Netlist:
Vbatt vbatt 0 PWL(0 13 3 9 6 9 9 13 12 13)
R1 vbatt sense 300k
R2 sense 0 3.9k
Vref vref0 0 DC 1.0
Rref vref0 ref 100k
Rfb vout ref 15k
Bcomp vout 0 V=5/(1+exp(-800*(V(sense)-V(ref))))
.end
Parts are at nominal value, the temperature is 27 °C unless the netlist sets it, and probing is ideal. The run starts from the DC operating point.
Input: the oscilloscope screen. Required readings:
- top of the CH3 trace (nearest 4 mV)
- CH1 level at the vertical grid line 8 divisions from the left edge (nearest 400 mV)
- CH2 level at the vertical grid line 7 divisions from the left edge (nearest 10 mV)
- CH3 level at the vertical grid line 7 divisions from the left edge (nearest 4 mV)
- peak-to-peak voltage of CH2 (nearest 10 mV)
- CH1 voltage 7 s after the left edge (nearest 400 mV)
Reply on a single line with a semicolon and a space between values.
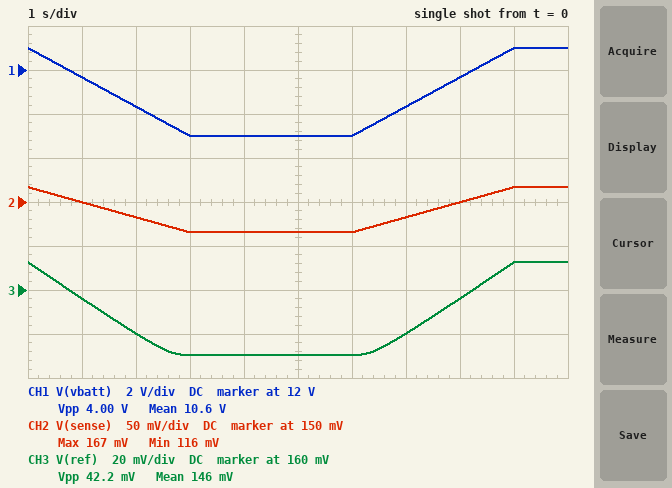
172 mV; 11.6 V; 130 mV; 140 mV; 50 mV; 10.4 V
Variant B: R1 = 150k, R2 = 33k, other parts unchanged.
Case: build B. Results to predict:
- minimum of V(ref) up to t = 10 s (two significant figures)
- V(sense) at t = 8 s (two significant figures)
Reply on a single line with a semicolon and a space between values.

1.6 V; 2.1 V
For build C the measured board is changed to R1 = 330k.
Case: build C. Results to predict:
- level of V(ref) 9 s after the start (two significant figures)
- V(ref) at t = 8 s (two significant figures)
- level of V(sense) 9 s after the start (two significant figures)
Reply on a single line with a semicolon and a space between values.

160 mV; 140 mV; 150 mV
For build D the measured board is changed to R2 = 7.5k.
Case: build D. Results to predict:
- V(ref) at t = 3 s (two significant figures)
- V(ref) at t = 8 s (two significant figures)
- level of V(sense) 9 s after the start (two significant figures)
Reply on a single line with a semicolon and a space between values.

220 mV; 290 mV; 320 mV
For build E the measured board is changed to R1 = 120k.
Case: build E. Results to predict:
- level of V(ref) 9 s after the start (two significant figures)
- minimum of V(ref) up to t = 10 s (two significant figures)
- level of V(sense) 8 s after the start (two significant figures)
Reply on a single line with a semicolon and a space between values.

410 mV; 290 mV; 370 mV
